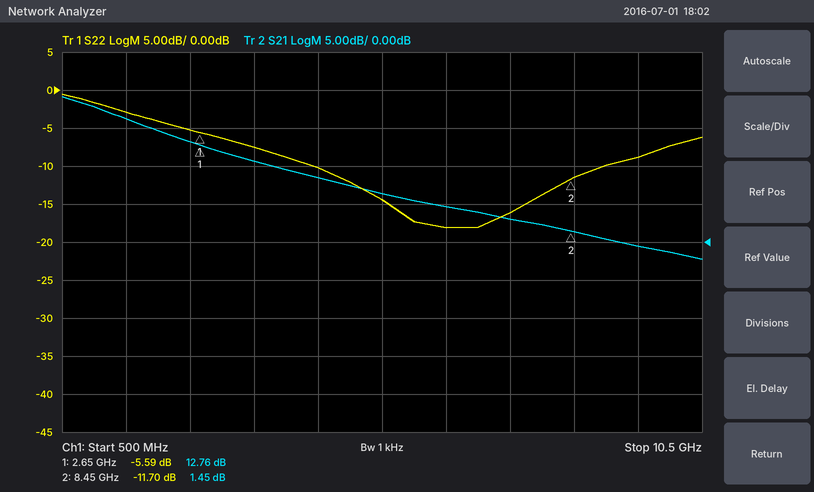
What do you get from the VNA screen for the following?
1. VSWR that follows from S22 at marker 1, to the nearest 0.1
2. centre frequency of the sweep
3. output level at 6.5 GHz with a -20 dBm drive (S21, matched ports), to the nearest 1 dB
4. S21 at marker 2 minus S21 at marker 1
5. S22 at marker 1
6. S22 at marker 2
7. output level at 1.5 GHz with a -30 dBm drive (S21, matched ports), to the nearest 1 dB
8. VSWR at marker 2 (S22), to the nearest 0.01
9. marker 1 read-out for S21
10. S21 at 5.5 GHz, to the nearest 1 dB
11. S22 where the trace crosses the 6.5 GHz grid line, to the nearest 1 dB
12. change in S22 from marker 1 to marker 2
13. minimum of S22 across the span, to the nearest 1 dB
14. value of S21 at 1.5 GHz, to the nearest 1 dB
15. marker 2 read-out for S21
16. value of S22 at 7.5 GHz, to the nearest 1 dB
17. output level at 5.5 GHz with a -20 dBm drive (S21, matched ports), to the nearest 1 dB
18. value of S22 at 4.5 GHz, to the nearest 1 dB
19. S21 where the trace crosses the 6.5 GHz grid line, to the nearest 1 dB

3.2
5.5 GHz
-15 dBm
-11.31 dB
-5.59 dB
-11.70 dB
-14 dBm
1.70
12.76 dB
6 dB
-18 dB
-6.11 dB
-18 dB
16 dB
1.45 dB
-16 dB
-14 dBm
-10 dB
5 dB
